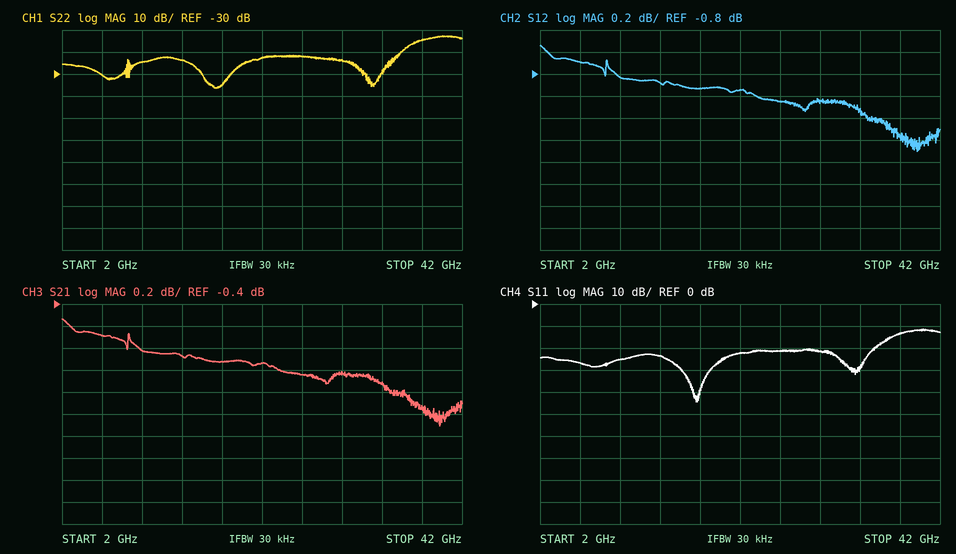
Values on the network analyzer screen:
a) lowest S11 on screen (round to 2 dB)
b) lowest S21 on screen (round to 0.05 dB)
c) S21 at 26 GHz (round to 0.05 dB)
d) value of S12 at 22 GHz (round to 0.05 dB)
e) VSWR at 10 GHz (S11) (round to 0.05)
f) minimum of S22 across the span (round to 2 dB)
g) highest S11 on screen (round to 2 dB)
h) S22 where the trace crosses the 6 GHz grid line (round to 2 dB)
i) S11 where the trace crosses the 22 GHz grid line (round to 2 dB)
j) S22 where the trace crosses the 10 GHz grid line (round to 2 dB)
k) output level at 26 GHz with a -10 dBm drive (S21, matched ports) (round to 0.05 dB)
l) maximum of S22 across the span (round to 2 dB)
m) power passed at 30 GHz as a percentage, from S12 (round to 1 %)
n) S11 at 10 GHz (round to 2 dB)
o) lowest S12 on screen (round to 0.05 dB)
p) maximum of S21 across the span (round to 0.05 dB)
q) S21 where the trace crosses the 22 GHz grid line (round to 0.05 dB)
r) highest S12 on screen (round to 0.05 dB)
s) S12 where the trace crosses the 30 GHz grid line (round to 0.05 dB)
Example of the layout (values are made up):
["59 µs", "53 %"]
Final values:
["-44 dB", "-1.50 dB", "-1.05 dB", "-0.95 dB", "1.10", "-36 dB", "-12 dB", "-30 dB", "-22 dB", "-24 dB", "-11.05 dBm", "-12 dB", "79 %", "-26 dB", "-1.50 dB", "-0.55 dB", "-0.95 dB", "-0.55 dB", "-1.05 dB"]
